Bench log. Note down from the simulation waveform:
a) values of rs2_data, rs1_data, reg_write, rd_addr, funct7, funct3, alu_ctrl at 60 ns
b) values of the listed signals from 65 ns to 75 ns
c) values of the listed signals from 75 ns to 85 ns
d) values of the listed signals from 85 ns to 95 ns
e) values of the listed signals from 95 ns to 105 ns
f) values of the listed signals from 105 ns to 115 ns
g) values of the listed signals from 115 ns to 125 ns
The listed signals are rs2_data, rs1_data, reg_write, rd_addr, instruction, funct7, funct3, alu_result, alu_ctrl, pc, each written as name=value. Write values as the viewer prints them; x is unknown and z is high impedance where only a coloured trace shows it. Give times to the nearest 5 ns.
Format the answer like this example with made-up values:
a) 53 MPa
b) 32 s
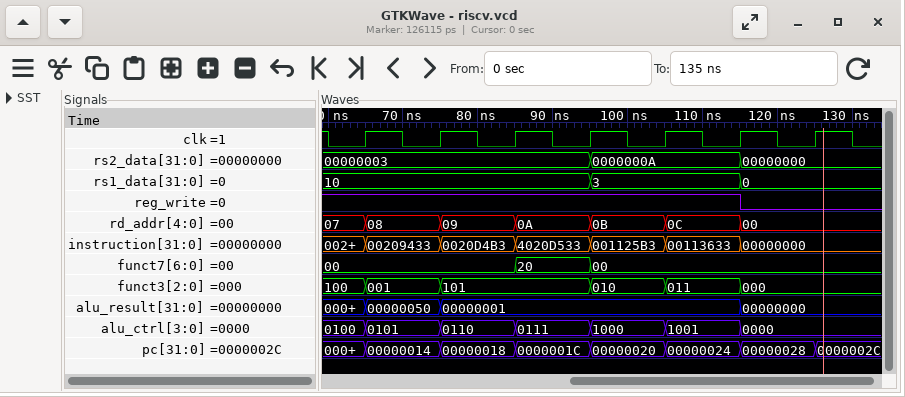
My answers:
a) rs2_data=00000003, rs1_data=10, reg_write=1, rd_addr=07, funct7=00, funct3=100, alu_ctrl=0100
b) rs2_data=00000003, rs1_data=10, reg_write=1, rd_addr=08, instruction=00209433, funct7=00, funct3=001, alu_result=00000050, alu_ctrl=0101, pc=00000014
c) rs2_data=00000003, rs1_data=10, reg_write=1, rd_addr=09, instruction=0020D4B3, funct7=00, funct3=101, alu_result=00000001, alu_ctrl=0110, pc=00000018
d) rs2_data=00000003, rs1_data=10, reg_write=1, rd_addr=0A, instruction=4020D533, funct7=20, funct3=101, alu_result=00000001, alu_ctrl=0111, pc=0000001C
e) rs2_data=0000000A, rs1_data=3, reg_write=1, rd_addr=0B, instruction=001125B3, funct7=00, funct3=010, alu_result=00000001, alu_ctrl=1000, pc=00000020
f) rs2_data=0000000A, rs1_data=3, reg_write=1, rd_addr=0C, instruction=00113633, funct7=00, funct3=011, alu_result=00000001, alu_ctrl=1001, pc=00000024
g) rs2_data=00000000, rs1_data=0, reg_write=0, rd_addr=00, instruction=00000000, funct7=00, funct3=000, alu_result=00000000, alu_ctrl=0000, pc=00000028
